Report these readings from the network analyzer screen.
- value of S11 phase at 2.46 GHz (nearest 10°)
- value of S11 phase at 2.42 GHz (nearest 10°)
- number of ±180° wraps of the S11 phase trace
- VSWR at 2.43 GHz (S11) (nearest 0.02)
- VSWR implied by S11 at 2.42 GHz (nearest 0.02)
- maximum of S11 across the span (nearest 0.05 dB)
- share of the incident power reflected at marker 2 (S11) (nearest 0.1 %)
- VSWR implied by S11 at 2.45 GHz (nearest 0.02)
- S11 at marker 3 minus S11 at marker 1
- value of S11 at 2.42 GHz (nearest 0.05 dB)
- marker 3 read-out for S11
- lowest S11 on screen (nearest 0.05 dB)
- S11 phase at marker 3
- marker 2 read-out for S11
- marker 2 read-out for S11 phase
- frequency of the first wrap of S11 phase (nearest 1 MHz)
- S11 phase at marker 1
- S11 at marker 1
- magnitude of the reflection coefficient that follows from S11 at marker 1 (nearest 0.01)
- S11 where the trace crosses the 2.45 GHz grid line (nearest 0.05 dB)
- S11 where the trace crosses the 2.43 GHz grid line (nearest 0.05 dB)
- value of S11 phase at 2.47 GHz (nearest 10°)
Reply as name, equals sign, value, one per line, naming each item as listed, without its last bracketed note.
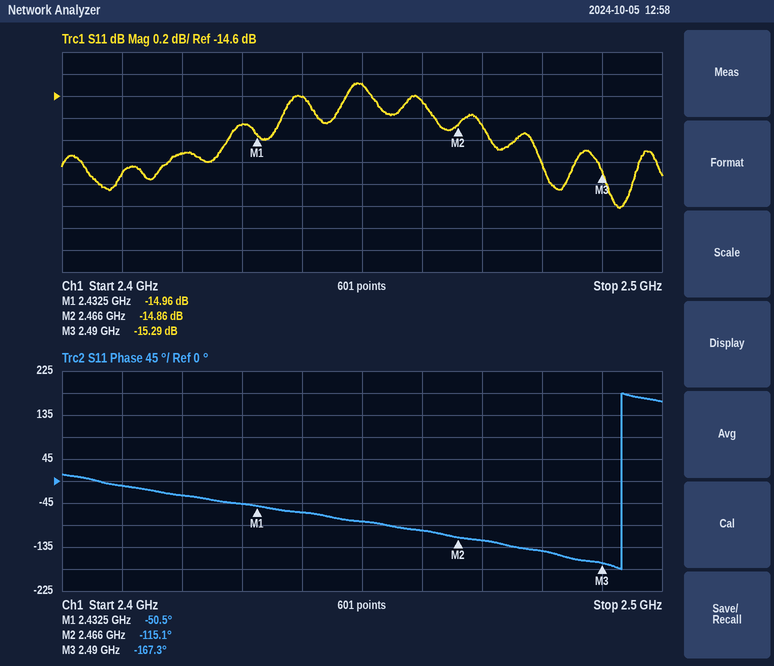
value of S11 phase at 2.46 GHz = -100°
value of S11 phase at 2.42 GHz = -30°
number of ±180° wraps of the S11 phase trace = 1
VSWR at 2.43 GHz (S11) = 1.44
VSWR implied by S11 at 2.42 GHz = 1.42
maximum of S11 across the span = -14.50 dB
share of the incident power reflected at marker 2 (S11) = 3.3 %
VSWR implied by S11 at 2.45 GHz = 1.46
S11 at marker 3 minus S11 at marker 1 = -0.33 dB
value of S11 at 2.42 GHz = -15.10 dB
marker 3 read-out for S11 = -15.29 dB
lowest S11 on screen = -15.60 dB
S11 phase at marker 3 = -167.3°
marker 2 read-out for S11 = -14.86 dB
marker 2 read-out for S11 phase = -115.1°
frequency of the first wrap of S11 phase = 2.493 GHz
S11 phase at marker 1 = -50.5°
S11 at marker 1 = -14.96 dB
magnitude of the reflection coefficient that follows from S11 at marker 1 = 0.18
S11 where the trace crosses the 2.45 GHz grid line = -14.50 dB
S11 where the trace crosses the 2.43 GHz grid line = -14.85 dB
value of S11 phase at 2.47 GHz = -120°
